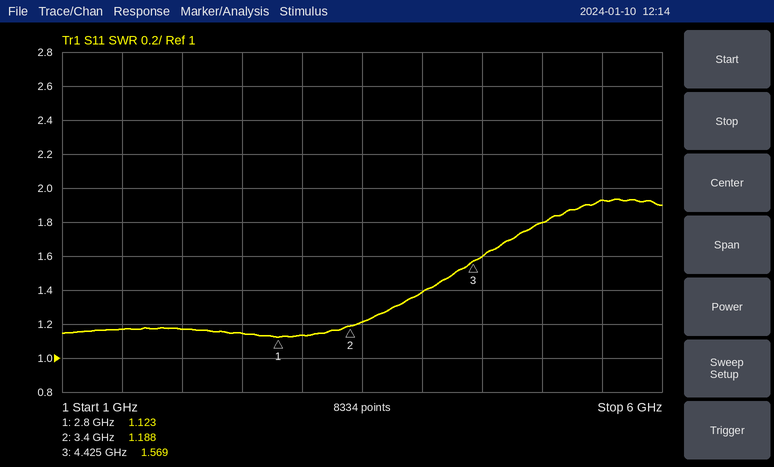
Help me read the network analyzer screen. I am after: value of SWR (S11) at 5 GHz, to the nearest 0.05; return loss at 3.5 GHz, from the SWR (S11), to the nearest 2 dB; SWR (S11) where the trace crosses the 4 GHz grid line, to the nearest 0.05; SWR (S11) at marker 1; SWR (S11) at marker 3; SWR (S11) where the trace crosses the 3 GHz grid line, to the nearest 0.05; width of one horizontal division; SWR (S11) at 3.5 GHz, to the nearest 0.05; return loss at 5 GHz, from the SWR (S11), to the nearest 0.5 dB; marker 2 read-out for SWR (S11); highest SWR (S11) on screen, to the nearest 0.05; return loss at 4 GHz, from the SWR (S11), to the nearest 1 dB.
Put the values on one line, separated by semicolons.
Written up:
1.80; 20 dB; 1.40; 1.123; 1.569; 1.15; 500 MHz; 1.20; 11.0 dB; 1.188; 1.95; 16 dB
